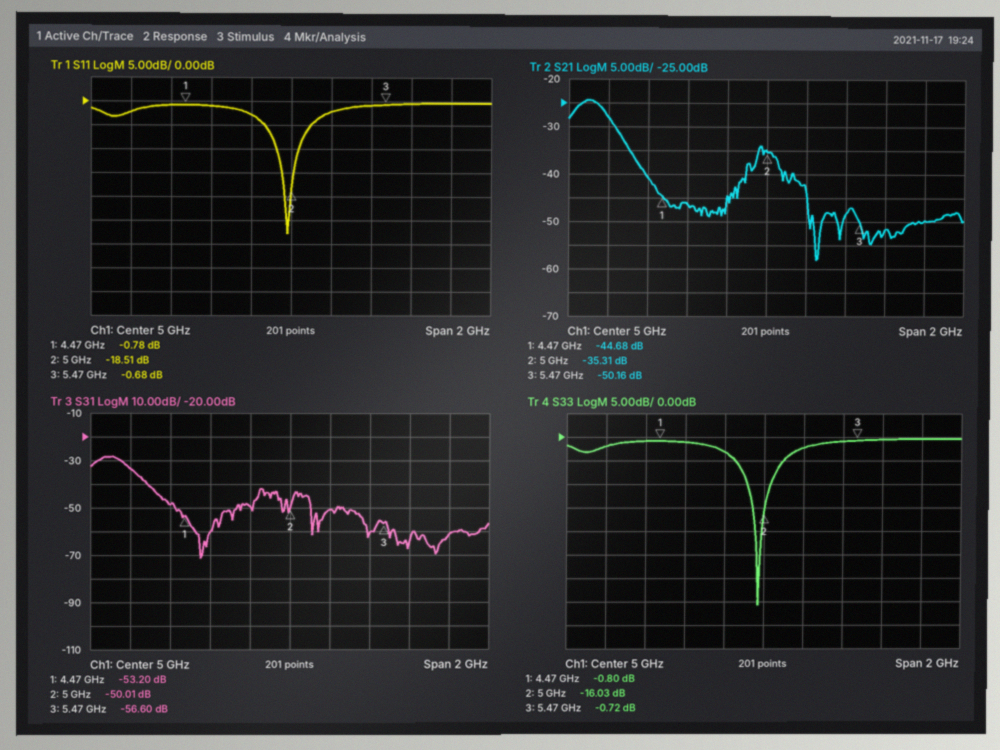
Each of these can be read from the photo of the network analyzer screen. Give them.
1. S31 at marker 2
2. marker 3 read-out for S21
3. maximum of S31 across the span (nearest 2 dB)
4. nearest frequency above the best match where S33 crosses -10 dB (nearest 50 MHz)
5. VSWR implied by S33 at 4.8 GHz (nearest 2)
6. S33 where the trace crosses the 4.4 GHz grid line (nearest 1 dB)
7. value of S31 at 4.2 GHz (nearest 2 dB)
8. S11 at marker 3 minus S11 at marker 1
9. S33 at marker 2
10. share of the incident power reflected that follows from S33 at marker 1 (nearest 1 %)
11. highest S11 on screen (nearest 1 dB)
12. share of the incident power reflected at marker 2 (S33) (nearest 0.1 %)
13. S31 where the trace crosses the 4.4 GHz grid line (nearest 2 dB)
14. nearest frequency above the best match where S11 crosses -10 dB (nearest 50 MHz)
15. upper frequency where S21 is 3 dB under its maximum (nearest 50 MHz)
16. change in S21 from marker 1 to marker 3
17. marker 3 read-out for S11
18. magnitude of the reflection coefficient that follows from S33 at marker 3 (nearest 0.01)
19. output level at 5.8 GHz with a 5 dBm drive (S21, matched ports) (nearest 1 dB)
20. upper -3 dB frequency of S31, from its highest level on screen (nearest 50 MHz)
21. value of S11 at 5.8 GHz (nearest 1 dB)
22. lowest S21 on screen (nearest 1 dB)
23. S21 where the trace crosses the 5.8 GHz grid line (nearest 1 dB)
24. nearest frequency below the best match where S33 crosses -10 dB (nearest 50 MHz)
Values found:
-50.01 dB
-50.16 dB
-28 dB
5.05 GHz
6
-1 dB
-34 dB
0.10 dB
-16.03 dB
83 %
0 dB
2.5 %
-48 dB
5.05 GHz
4.20 GHz
-5.48 dB
-0.68 dB
0.92
-45 dBm
4.15 GHz
0 dB
-58 dB
-50 dB
4.90 GHz
